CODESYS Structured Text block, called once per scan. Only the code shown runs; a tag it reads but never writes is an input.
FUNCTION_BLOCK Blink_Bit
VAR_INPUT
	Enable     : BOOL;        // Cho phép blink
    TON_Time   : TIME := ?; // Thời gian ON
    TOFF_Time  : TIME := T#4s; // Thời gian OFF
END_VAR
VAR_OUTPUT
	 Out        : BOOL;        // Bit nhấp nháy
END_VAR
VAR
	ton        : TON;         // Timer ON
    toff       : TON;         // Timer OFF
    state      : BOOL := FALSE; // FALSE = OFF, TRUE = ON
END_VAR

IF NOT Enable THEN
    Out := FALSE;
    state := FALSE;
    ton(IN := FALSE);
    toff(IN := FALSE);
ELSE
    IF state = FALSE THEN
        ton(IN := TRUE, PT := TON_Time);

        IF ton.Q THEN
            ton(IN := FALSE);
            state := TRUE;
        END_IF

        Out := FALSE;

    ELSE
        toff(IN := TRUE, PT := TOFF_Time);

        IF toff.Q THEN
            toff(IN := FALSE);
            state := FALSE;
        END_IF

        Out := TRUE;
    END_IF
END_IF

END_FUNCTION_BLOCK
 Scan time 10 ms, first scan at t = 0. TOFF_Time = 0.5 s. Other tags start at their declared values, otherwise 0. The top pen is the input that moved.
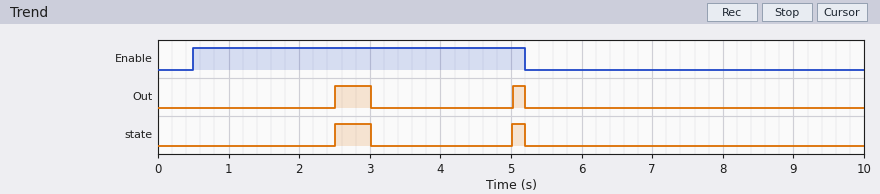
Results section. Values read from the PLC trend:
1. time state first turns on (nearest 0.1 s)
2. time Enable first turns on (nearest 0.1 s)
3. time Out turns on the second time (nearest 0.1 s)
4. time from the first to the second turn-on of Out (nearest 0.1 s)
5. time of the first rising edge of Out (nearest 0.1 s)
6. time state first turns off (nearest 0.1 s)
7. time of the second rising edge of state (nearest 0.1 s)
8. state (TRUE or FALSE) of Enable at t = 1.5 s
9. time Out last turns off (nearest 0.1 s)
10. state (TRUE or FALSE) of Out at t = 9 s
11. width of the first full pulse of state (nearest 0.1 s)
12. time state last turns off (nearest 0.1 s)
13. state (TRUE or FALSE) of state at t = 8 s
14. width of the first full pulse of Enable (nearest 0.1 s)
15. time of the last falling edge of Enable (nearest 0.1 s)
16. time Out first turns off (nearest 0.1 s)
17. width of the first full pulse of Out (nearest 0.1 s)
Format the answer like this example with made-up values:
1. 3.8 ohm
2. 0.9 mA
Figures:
1. 2.5 s
2. 0.5 s
3. 5.0 s
4. 2.5 s
5. 2.5 s
6. 3.0 s
7. 5.0 s
8. TRUE
9. 5.2 s
10. FALSE
11. 0.5 s
12. 5.2 s
13. FALSE
14. 4.7 s
15. 5.2 s
16. 3.0 s
17. 0.5 s
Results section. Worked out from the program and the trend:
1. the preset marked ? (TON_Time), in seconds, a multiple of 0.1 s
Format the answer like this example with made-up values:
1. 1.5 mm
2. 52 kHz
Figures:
1. 2.0 s
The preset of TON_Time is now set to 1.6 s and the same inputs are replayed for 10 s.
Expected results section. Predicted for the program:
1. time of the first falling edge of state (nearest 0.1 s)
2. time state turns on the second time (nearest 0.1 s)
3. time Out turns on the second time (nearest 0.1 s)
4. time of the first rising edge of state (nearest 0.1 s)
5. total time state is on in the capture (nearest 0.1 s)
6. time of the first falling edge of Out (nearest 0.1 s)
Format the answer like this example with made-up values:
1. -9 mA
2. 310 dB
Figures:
1. 2.6 s
2. 4.2 s
3. 4.2 s
4. 2.1 s
5. 1.0 s
6. 2.6 s
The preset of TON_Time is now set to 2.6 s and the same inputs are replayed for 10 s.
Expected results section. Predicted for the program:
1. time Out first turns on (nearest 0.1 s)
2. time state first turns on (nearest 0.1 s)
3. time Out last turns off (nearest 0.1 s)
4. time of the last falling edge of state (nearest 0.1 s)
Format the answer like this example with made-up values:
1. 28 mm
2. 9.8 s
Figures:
1. 3.1 s
2. 3.1 s
3. 3.6 s
4. 3.6 s
